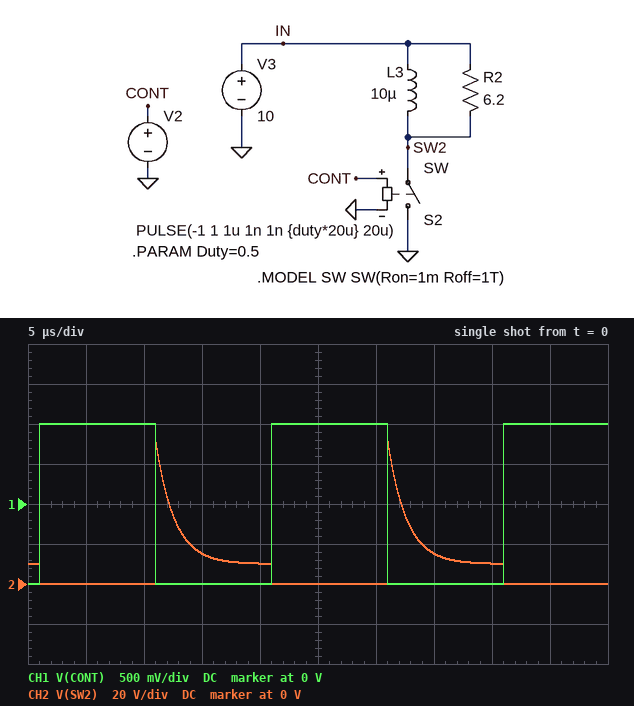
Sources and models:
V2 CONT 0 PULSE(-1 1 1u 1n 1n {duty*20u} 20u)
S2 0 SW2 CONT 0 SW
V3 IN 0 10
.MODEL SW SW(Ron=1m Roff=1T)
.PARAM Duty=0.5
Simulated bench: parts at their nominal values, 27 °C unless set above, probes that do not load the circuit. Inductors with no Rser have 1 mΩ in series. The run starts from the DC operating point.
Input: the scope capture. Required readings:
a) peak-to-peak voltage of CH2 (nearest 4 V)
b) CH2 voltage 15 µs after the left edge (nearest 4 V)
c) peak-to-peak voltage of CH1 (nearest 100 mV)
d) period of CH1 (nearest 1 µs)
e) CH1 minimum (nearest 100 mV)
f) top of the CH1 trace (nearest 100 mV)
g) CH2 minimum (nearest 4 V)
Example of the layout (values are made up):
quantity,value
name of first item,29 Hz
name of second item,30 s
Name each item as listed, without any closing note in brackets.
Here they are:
quantity,value
peak-to-peak voltage of CH2,72 V
CH2 voltage 15 µs after the left edge,16 V
peak-to-peak voltage of CH1,2.0 V
period of CH1,20 µs
CH1 minimum,-1.0 V
top of the CH1 trace,1.0 V
CH2 minimum,0 V
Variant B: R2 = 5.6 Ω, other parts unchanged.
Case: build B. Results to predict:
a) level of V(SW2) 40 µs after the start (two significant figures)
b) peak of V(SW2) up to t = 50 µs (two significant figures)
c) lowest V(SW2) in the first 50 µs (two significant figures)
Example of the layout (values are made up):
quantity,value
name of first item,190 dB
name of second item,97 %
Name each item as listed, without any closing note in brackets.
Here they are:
quantity,value
level of V(SW2) 40 µs after the start,10 V
peak of V(SW2) up to t = 50 µs,66 V
lowest V(SW2) in the first 50 µs,1.8 mV
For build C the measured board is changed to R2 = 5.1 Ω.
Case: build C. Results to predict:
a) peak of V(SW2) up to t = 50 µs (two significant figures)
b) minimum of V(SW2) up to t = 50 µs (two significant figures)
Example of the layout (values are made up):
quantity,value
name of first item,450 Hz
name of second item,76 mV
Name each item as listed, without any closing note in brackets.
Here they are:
quantity,value
peak of V(SW2) up to t = 50 µs,61 V
minimum of V(SW2) up to t = 50 µs,2.0 mV
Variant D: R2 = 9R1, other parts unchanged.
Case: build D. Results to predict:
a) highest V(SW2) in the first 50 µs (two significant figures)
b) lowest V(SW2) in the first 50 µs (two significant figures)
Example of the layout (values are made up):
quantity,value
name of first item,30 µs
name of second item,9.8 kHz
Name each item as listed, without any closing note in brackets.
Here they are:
quantity,value
highest V(SW2) in the first 50 µs,100 V
lowest V(SW2) in the first 50 µs,1.1 mV
